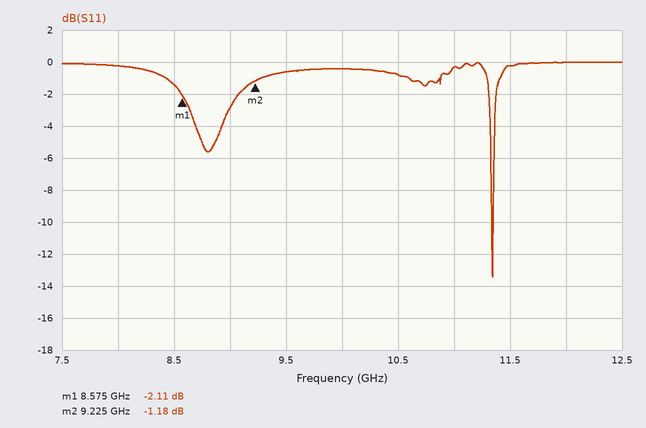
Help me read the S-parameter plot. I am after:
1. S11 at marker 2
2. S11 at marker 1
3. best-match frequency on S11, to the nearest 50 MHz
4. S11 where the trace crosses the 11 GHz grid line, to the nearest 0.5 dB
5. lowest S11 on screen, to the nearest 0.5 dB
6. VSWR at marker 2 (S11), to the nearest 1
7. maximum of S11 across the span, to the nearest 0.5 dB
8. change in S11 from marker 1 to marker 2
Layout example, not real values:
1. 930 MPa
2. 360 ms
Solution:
1. -1.18 dB
2. -2.11 dB
3. 11.35 GHz
4. -0.5 dB
5. -13.5 dB
6. 15
7. 0.0 dB
8. 0.93 dB
